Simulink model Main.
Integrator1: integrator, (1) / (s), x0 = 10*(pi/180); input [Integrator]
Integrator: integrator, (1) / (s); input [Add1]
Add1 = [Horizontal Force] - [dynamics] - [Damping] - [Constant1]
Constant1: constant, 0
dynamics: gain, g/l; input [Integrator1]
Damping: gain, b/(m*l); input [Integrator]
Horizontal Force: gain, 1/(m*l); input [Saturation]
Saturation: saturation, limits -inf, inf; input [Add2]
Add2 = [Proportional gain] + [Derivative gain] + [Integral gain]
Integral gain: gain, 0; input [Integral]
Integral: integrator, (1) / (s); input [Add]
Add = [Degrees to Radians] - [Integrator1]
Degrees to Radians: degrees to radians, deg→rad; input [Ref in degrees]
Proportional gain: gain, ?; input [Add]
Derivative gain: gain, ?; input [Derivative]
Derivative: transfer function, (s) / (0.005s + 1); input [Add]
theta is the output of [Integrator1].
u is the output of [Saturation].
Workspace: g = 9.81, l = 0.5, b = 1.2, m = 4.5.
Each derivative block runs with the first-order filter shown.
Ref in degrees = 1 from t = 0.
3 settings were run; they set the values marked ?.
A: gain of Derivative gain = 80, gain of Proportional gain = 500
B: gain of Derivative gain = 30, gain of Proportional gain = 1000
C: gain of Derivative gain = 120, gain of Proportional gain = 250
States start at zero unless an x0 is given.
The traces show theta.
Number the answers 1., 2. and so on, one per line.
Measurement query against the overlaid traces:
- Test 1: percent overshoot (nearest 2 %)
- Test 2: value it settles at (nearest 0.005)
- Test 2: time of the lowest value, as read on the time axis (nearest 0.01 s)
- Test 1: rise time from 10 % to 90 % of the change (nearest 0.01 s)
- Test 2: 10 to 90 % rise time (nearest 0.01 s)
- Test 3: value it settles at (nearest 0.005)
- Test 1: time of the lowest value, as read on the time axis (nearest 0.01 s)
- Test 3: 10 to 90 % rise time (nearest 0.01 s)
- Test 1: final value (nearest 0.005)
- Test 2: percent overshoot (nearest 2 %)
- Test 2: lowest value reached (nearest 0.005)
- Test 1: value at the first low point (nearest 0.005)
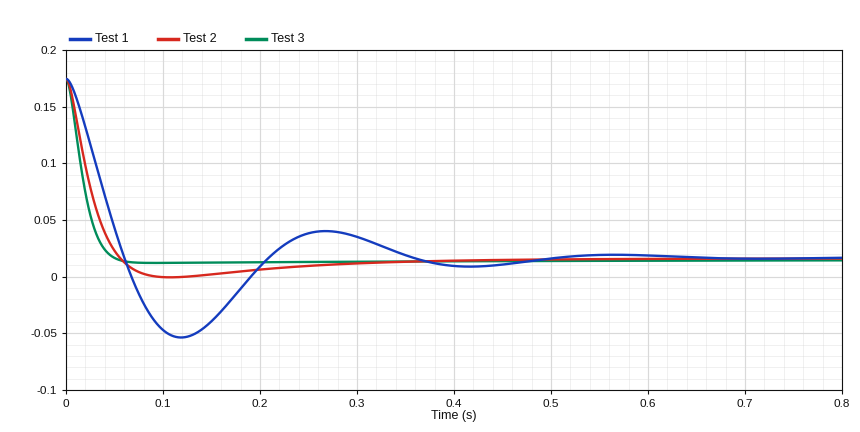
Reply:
1. 44 %
2. 0.015
3. 0.11 s
4. 0.04 s
5. 0.04 s
6. 0.015
7. 0.12 s
8. 0.03 s
9. 0.015
10. 10 %
11. 0.000
12. -0.055
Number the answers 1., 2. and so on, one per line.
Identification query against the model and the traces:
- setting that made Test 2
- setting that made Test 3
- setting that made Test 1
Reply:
1. A
2. C
3. B
